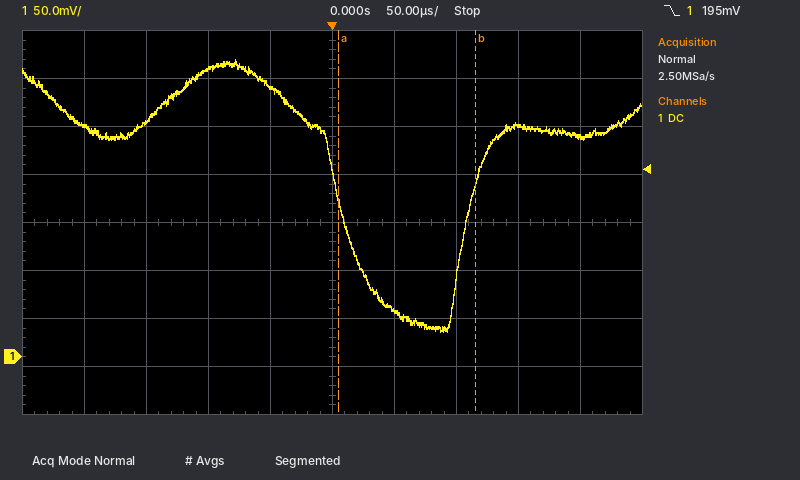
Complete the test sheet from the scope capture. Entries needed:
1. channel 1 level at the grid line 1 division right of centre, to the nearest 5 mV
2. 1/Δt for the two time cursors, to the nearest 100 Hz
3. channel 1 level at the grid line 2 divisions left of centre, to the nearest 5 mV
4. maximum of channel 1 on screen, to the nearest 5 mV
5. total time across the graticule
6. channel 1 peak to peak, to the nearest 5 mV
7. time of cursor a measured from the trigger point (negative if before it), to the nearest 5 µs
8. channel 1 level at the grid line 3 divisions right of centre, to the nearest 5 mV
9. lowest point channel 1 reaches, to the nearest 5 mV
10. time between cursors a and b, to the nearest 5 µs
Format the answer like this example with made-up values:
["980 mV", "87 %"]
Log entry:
["50 mV", "9.1 kHz", "300 mV", "310 mV", "500 µs", "285 mV", "+5 µs", "240 mV", "25 mV", "110 µs"]
